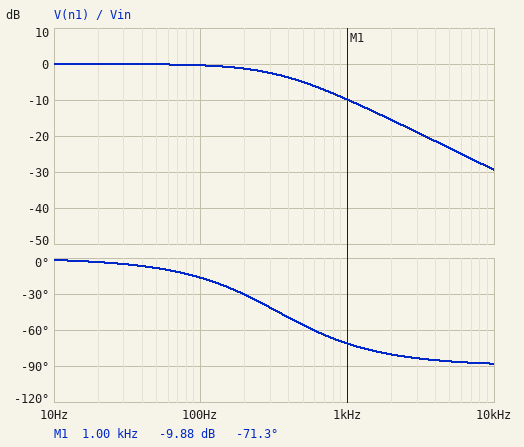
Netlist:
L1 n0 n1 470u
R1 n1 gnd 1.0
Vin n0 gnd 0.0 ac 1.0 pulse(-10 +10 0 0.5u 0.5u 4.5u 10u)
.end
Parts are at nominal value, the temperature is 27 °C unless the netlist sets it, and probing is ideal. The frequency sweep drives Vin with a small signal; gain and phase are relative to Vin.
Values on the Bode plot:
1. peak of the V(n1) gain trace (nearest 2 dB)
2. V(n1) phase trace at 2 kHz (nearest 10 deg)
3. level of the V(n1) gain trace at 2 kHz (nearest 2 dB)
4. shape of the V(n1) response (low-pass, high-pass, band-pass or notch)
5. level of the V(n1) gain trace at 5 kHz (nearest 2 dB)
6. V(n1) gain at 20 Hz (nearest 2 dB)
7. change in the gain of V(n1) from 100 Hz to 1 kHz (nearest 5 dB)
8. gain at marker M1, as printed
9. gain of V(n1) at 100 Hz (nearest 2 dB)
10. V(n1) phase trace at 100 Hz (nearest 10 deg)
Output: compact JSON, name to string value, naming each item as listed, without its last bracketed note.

{"peak of the V(n1) gain trace": "0 dB", "V(n1) phase trace at 2 kHz": "-80 deg", "level of the V(n1) gain trace at 2 kHz": "-16 dB", "shape of the V(n1) response": "low-pass", "level of the V(n1) gain trace at 5 kHz": "-24 dB", "V(n1) gain at 20 Hz": "0 dB", "change in the gain of V(n1) from 100 Hz to 1 kHz": "-10 dB", "gain at marker M1, as printed": "-9.88 dB", "gain of V(n1) at 100 Hz": "0 dB", "V(n1) phase trace at 100 Hz": "-20 deg"}
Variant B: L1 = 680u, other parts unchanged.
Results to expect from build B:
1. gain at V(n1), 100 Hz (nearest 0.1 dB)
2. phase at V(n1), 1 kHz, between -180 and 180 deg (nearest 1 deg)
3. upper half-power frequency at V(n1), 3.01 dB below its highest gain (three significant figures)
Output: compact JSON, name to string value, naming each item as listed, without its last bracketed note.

{"gain at V(n1), 100 Hz": "-0.7 dB", "phase at V(n1), 1 kHz, between -180 and 180 deg": "-77 deg", "upper half-power frequency at V(n1), 3.01 dB below its highest gain": "234 Hz"}
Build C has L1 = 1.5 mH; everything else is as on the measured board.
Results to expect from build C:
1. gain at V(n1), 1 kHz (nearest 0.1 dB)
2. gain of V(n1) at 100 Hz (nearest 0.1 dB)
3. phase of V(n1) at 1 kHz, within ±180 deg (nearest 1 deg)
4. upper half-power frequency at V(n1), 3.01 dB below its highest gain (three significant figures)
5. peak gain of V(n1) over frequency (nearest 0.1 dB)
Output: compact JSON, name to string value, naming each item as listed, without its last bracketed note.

{"gain at V(n1), 1 kHz": "-19.5 dB", "gain of V(n1) at 100 Hz": "-2.8 dB", "phase of V(n1) at 1 kHz, within ±180 deg": "-84 deg", "upper half-power frequency at V(n1), 3.01 dB below its highest gain": "106 Hz", "peak gain of V(n1) over frequency": "0 dB"}
